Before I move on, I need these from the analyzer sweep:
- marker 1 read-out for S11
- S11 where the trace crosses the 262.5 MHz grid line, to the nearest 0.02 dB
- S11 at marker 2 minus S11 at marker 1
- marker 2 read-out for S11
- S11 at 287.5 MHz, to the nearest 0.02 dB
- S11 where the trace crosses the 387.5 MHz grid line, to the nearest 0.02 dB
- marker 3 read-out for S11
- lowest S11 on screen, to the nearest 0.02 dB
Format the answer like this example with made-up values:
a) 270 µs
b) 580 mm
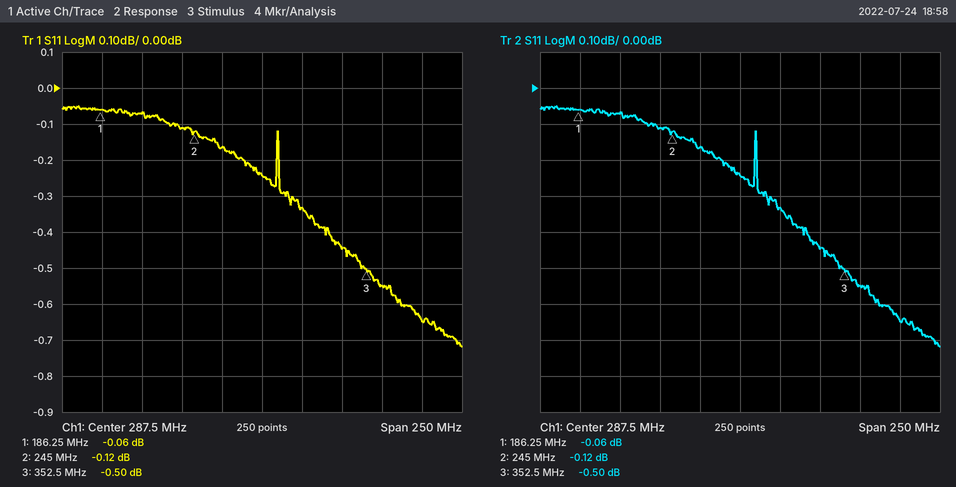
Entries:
a) -0.06 dB
b) -0.16 dB
c) -0.06 dB
d) -0.12 dB
e) -0.24 dB
f) -0.64 dB
g) -0.50 dB
h) -0.72 dB
